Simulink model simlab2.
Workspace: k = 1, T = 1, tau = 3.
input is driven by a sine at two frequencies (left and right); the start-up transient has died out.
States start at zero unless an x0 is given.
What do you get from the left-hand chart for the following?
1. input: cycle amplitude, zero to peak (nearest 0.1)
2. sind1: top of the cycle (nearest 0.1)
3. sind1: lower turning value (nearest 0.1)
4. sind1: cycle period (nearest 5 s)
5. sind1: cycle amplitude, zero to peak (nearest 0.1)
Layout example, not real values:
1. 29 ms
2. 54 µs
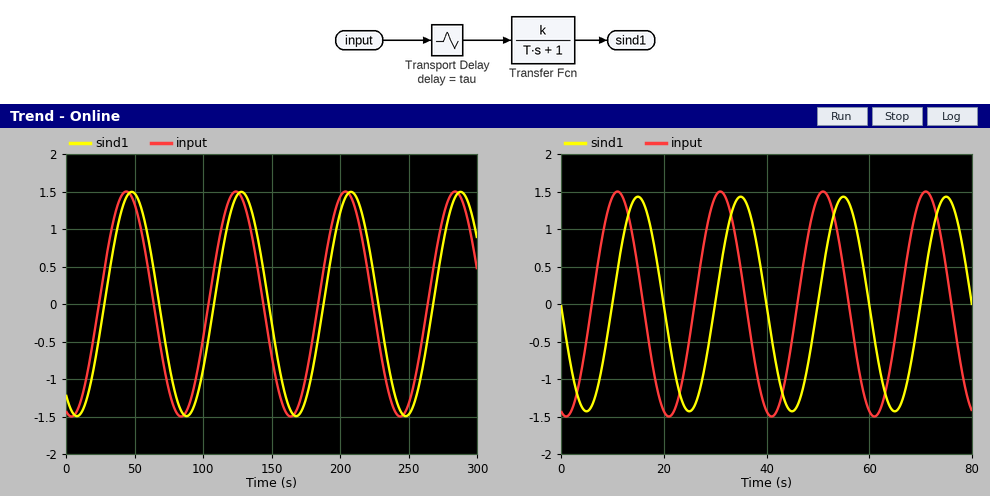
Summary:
1. 1.5
2. 1.5
3. -1.5
4. 80 s
5. 1.5
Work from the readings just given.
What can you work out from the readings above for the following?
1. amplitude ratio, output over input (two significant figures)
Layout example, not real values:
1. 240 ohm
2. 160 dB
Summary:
1. 1.0
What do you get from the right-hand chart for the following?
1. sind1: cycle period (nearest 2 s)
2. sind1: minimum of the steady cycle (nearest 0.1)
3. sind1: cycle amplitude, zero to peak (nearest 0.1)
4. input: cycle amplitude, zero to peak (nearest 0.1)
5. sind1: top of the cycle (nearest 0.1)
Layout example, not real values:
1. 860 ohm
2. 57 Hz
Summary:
1. 20 s
2. -1.4
3. 1.4
4. 1.5
5. 1.4
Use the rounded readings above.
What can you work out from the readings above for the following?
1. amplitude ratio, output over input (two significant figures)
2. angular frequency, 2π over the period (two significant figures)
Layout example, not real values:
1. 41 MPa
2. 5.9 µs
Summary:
1. 0.93
2. 0.31 rad/s
